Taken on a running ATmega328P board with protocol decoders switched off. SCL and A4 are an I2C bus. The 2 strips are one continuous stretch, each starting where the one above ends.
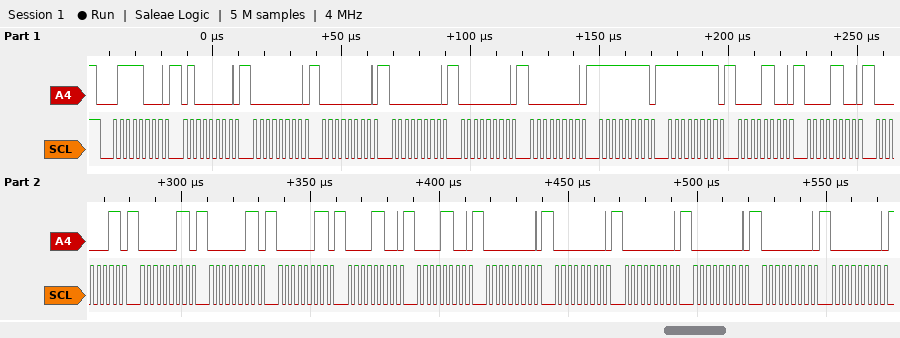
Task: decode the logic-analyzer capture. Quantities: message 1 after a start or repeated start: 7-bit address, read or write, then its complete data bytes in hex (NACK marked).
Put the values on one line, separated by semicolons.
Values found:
0x3C write: 40 00 00 00 00 00 FF FF 0C 0C 03 03 03 03 0C 0C 00 00 00 00 00 00
